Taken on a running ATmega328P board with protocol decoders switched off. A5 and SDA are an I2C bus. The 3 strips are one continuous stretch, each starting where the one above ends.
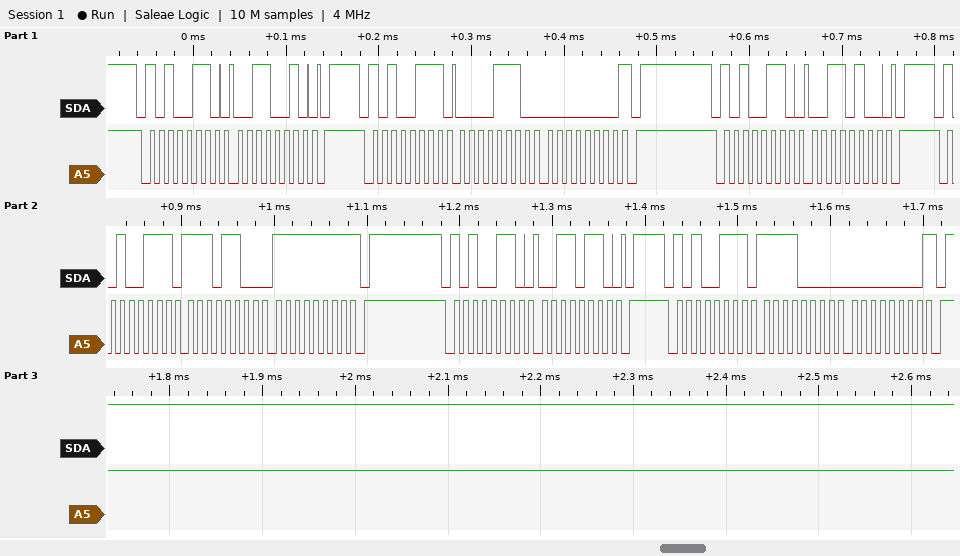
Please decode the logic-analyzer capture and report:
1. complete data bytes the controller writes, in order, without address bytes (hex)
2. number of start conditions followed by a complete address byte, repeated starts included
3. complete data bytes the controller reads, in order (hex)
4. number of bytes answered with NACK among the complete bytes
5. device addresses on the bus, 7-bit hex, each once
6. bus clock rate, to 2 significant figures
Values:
32 34 36
6
0E 00 EC FF F0 00
3
0x53
100 kHz
